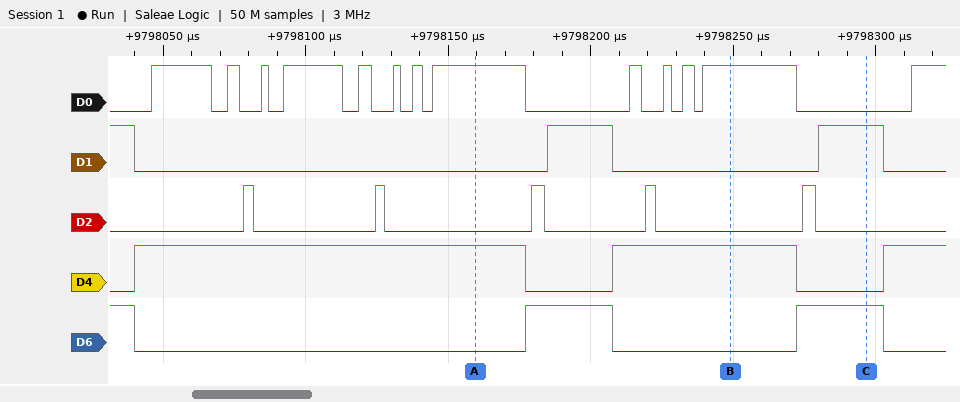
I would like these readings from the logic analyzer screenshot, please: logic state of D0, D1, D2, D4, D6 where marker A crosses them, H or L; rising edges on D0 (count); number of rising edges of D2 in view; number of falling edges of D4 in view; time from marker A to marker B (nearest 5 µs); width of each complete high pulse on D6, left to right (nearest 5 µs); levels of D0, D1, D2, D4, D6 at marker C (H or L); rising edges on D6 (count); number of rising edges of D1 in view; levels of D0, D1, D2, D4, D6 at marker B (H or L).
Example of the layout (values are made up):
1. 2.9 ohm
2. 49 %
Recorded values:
1. D0=H, D1=L, D2=L, D4=H, D6=L
2. 13
3. 5
4. 2
5. 90 µs
6. 30 µs, 30 µs
7. D0=L, D1=H, D2=L, D4=L, D6=H
8. 2
9. 2
10. D0=H, D1=L, D2=L, D4=H, D6=L
